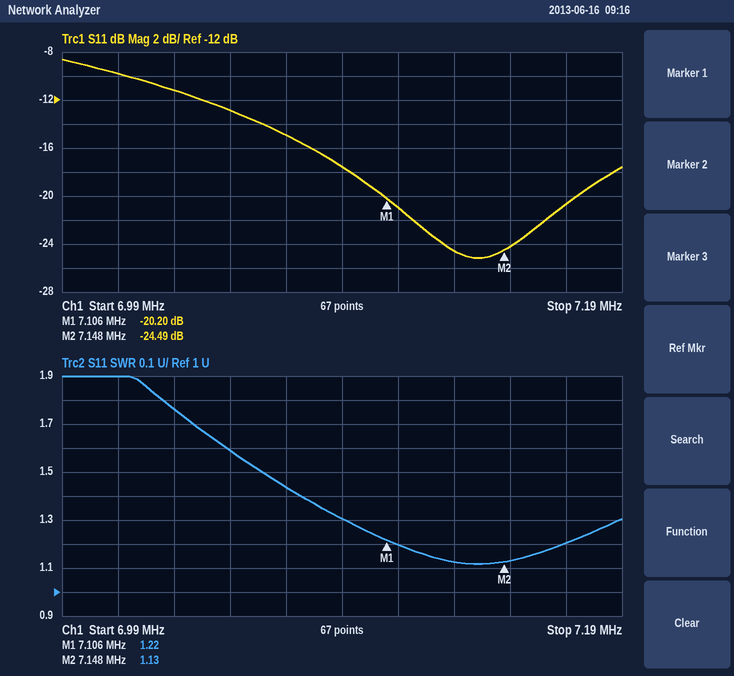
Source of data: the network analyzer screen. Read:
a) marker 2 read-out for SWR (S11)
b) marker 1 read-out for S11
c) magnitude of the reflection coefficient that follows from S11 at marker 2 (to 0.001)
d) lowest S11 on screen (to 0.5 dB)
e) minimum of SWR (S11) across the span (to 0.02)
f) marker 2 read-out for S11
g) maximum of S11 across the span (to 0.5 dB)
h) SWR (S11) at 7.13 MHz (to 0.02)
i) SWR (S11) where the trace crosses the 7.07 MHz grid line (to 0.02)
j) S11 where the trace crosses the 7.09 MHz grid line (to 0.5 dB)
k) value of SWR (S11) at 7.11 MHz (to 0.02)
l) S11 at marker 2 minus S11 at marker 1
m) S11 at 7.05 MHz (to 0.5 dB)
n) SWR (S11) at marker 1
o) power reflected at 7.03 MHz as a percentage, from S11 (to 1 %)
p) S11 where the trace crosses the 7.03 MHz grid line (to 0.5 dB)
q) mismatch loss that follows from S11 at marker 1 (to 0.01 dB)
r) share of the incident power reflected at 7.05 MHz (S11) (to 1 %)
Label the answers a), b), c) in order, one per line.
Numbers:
a) 1.13
b) -20.20 dB
c) 0.060
d) -25.0 dB
e) 1.12
f) -24.49 dB
g) -8.5 dB
h) 1.12
i) 1.44
j) -17.5 dB
k) 1.20
l) -4.29 dB
m) -13.0 dB
n) 1.22
o) 8 %
p) -11.0 dB
q) 0.04 dB
r) 5 %
